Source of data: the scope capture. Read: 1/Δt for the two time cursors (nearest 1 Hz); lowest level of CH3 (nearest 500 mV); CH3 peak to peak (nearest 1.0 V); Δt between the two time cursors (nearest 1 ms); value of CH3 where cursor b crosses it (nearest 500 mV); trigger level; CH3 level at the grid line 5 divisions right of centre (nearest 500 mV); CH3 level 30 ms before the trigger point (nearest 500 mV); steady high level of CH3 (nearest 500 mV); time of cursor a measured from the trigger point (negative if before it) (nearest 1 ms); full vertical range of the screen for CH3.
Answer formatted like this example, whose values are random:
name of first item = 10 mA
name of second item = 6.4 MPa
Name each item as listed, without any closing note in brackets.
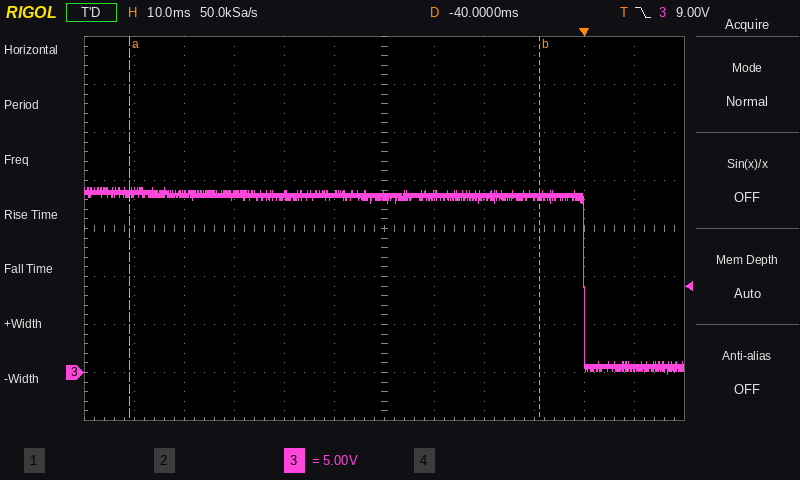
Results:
1/Δt for the two time cursors = 12 Hz
lowest level of CH3 = 0.0 V
CH3 peak to peak = 19.0 V
Δt between the two time cursors = 82 ms
value of CH3 where cursor b crosses it = 18.5 V
trigger level = 9.00 V
CH3 level at the grid line 5 divisions right of centre = 500 mV
CH3 level 30 ms before the trigger point = 18.5 V
steady high level of CH3 = 18.5 V
time of cursor a measured from the trigger point (negative if before it) = -91 ms
full vertical range of the screen for CH3 = 40 V
